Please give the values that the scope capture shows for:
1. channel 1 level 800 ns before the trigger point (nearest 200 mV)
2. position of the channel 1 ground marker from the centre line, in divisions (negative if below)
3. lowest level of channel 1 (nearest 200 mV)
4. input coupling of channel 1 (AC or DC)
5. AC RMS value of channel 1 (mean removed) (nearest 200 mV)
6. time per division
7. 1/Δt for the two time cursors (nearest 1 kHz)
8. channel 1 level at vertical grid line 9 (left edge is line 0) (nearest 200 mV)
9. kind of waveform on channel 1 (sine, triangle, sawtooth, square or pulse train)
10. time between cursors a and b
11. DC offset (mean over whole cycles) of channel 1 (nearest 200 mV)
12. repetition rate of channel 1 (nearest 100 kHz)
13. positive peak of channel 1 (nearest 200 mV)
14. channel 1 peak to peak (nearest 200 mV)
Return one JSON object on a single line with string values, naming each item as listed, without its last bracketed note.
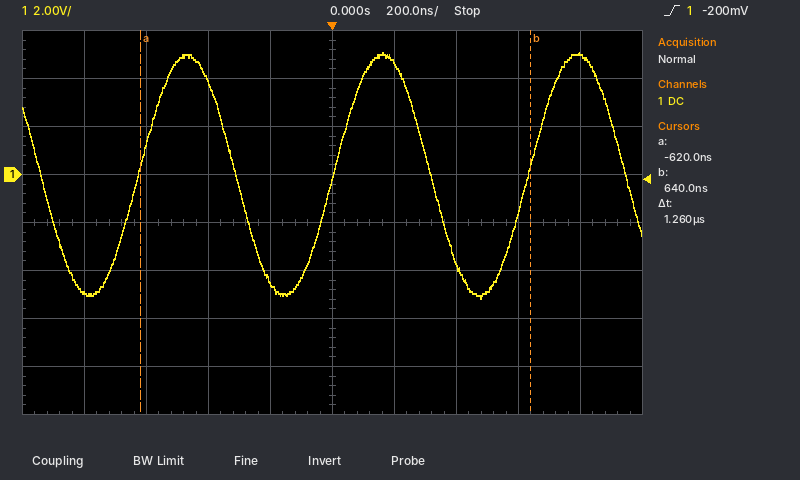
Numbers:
{"channel 1 level 800 ns before the trigger point": "-5.0 V", "position of the channel 1 ground marker from the centre line, in divisions": "+1.0 div", "lowest level of channel 1": "-5.2 V", "input coupling of channel 1": "DC", "AC RMS value of channel 1 (mean removed)": "3.6 V", "time per division": "200 ns", "1/Δt for the two time cursors": "794 kHz", "channel 1 level at vertical grid line 9 (left edge is line 0)": "5.0 V", "kind of waveform on channel 1": "sine", "time between cursors a and b": "1.26 µs", "DC offset (mean over whole cycles) of channel 1": "0.0 V", "repetition rate of channel 1": "1.6 MHz", "positive peak of channel 1": "5.0 V", "channel 1 peak to peak": "10.2 V"}
